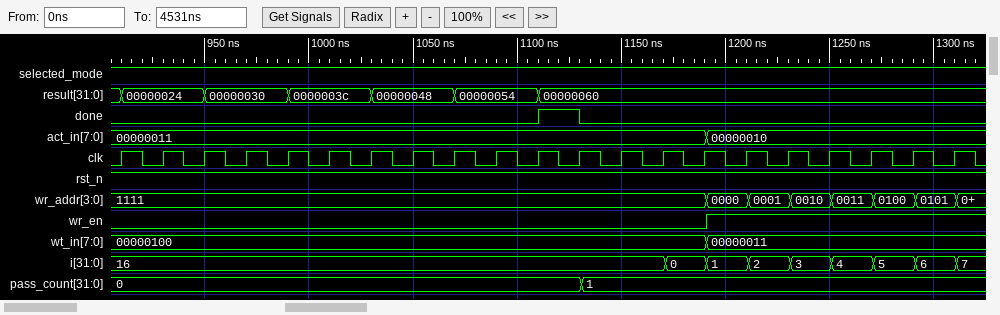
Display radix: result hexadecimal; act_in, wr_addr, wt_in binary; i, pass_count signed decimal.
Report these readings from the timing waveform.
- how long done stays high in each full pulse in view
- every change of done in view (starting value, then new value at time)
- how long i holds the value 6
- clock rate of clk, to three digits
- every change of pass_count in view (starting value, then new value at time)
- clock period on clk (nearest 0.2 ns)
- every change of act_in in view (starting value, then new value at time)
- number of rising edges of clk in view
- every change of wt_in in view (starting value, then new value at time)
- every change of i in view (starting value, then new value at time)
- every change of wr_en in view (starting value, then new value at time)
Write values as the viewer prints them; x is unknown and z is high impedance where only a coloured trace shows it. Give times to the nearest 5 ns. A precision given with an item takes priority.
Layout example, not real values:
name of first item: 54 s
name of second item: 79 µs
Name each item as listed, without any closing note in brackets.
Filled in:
how long done stays high in each full pulse in view: 20 ns
every change of done in view: 0, 1 at 1110 ns, 0 at 1130 ns
how long i holds the value 6: 20 ns
clock rate of clk, to three digits: 50.0 MHz
every change of pass_count in view: 0, 1 at 1130 ns
clock period on clk: 20 ns
every change of act_in in view: 00000011, 00000010 at 1190 ns
number of rising edges of clk in view: 21
every change of wt_in in view: 00000100, 00000011 at 1190 ns
every change of i in view: 16, 0 at 1170 ns, 1 at 1190 ns, 2 at 1210 ns, 3 at 1230 ns, 4 at 1250 ns, 5 at 1270 ns, 6 at 1290 ns, 7 at 1310 ns
every change of wr_en in view: 0, 1 at 1190 ns
